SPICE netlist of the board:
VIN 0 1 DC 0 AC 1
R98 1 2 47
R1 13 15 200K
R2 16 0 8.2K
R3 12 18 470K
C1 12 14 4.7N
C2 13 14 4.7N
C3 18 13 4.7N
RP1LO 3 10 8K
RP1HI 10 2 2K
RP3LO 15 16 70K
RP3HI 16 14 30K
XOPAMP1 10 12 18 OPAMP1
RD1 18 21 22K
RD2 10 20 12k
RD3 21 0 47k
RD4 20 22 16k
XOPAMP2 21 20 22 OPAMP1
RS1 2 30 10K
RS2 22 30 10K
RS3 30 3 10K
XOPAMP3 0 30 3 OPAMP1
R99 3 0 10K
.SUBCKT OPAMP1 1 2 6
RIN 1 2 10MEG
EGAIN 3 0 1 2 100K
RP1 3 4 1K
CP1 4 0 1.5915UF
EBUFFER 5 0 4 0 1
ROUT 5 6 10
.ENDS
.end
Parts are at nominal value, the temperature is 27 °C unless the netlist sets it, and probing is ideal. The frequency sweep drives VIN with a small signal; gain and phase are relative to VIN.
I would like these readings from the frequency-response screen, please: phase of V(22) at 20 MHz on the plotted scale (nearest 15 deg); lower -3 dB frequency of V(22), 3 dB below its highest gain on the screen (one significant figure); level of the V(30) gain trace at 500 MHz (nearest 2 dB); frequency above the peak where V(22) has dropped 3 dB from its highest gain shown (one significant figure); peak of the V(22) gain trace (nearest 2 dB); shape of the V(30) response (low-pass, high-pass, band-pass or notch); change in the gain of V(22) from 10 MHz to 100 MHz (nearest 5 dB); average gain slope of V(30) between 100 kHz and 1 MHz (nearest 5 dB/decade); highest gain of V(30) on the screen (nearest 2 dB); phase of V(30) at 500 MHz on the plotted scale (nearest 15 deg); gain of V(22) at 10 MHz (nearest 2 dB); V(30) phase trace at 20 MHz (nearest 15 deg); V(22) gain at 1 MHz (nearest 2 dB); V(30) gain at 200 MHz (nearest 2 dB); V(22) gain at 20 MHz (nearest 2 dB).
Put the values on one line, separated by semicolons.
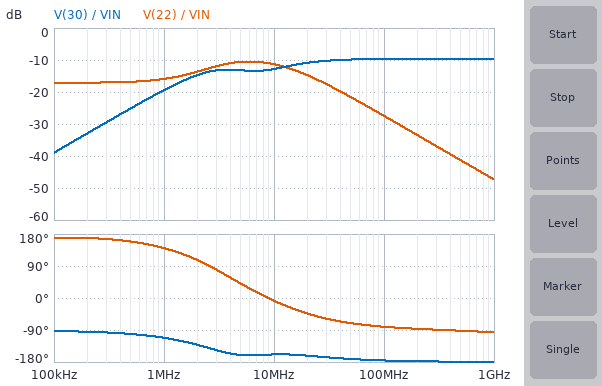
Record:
-45 deg; 2 MHz; -10 dB; 20 MHz; -10 dB; high-pass; -15 dB; 20 dB/decade; -10 dB; -180 deg; -12 dB; -165 deg; -16 dB; -10 dB; -14 dB
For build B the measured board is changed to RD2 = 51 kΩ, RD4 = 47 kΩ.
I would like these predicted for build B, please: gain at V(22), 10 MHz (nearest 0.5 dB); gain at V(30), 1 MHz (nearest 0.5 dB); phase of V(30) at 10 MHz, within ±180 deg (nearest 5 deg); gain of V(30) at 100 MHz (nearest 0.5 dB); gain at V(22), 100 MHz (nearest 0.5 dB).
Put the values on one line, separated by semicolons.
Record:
-12.0 dB; -19.0 dB; -165 deg; -9.5 dB; -28.5 dB
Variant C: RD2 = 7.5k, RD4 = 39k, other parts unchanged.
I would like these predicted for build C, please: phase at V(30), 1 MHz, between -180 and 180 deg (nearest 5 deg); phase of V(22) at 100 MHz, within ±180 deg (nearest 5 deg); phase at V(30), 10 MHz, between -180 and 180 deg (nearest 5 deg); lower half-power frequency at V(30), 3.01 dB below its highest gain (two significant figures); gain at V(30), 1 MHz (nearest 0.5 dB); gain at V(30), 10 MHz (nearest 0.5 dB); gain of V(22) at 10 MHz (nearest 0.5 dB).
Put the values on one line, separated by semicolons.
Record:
-90 deg; -85 deg; -140 deg; 10 MHz; -29.0 dB; -12.5 dB; -7.5 dB
